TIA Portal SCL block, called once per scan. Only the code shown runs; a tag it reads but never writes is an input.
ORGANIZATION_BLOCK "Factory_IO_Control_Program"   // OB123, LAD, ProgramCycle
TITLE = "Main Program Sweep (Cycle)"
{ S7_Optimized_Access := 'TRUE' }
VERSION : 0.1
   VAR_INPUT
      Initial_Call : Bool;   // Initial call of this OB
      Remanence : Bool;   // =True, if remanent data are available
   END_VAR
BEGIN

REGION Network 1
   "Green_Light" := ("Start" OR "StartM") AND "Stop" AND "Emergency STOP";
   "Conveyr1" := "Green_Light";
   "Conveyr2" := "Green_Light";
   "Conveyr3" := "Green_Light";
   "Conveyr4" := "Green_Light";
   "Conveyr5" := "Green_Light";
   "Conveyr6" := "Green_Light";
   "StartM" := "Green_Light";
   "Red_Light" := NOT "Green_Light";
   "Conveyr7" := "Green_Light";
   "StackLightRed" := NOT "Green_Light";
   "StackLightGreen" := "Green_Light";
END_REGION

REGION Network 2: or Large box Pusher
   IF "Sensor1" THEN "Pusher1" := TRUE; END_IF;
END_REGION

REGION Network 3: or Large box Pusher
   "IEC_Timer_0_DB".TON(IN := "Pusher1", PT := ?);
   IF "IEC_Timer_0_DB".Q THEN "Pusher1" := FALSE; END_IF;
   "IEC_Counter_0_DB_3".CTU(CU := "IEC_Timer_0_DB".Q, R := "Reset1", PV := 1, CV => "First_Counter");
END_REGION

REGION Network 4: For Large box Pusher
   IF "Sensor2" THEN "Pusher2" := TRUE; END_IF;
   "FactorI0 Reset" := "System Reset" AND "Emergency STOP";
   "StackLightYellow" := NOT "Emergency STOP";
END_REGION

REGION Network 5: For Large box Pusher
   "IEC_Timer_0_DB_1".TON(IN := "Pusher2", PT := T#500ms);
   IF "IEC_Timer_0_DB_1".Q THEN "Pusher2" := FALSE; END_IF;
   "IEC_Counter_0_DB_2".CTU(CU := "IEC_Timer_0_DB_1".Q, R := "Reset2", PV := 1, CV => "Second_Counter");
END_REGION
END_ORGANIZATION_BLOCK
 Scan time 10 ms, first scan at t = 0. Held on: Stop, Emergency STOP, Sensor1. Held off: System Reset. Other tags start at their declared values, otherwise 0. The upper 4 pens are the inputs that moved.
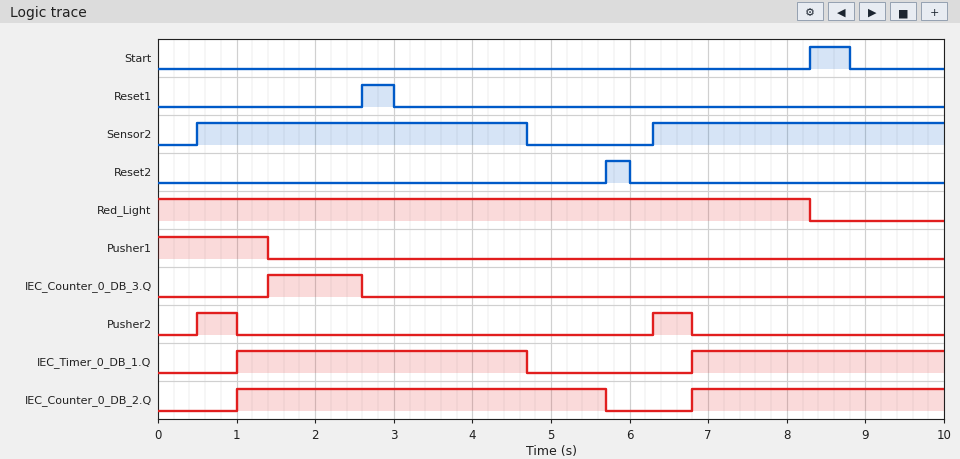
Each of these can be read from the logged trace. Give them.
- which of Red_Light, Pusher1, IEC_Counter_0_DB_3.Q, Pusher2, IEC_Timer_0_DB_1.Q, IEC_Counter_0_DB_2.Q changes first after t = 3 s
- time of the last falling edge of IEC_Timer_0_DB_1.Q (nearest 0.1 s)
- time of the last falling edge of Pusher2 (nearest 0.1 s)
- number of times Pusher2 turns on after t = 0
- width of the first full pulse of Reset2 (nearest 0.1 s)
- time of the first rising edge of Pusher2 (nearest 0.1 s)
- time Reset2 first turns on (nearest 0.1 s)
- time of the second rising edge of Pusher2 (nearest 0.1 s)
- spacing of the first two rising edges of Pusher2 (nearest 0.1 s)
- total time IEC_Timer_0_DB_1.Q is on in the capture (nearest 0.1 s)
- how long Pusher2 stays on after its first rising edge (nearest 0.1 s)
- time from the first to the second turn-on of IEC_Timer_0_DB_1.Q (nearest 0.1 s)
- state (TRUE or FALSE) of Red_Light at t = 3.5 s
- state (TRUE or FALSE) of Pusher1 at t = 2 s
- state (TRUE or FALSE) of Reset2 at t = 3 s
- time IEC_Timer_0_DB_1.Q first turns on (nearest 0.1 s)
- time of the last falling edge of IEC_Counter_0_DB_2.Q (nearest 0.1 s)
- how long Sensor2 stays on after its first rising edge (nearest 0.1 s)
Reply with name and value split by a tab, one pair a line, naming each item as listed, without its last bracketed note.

which of Red_Light, Pusher1, IEC_Counter_0_DB_3.Q, Pusher2, IEC_Timer_0_DB_1.Q, IEC_Counter_0_DB_2.Q changes first after t = 3 s	IEC_Timer_0_DB_1.Q
time of the last falling edge of IEC_Timer_0_DB_1.Q	4.7 s
time of the last falling edge of Pusher2	6.8 s
number of times Pusher2 turns on after t = 0	2
width of the first full pulse of Reset2	0.3 s
time of the first rising edge of Pusher2	0.5 s
time Reset2 first turns on	5.7 s
time of the second rising edge of Pusher2	6.3 s
spacing of the first two rising edges of Pusher2	5.8 s
total time IEC_Timer_0_DB_1.Q is on in the capture	6.9 s
how long Pusher2 stays on after its first rising edge	0.5 s
time from the first to the second turn-on of IEC_Timer_0_DB_1.Q	5.8 s
state (TRUE or FALSE) of Red_Light at t = 3.5 s	TRUE
state (TRUE or FALSE) of Pusher1 at t = 2 s	FALSE
state (TRUE or FALSE) of Reset2 at t = 3 s	FALSE
time IEC_Timer_0_DB_1.Q first turns on	1.0 s
time of the last falling edge of IEC_Counter_0_DB_2.Q	5.7 s
how long Sensor2 stays on after its first rising edge	4.2 s
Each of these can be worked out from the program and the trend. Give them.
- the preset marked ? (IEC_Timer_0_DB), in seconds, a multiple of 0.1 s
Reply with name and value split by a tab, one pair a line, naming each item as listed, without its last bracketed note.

the preset marked ? (IEC_Timer_0_DB), in seconds, a multiple of 0.1 s	1.4 s
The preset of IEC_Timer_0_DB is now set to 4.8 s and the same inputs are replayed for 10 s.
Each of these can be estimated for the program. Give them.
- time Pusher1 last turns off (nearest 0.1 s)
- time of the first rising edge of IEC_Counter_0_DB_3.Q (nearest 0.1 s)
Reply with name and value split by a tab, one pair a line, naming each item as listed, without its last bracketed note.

time Pusher1 last turns off	4.8 s
time of the first rising edge of IEC_Counter_0_DB_3.Q	4.8 s
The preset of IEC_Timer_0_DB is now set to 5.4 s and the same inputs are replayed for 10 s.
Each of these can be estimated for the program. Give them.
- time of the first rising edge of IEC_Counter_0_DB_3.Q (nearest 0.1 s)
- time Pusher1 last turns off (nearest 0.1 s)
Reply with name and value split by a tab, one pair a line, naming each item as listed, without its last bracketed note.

time of the first rising edge of IEC_Counter_0_DB_3.Q	5.4 s
time Pusher1 last turns off	5.4 s
